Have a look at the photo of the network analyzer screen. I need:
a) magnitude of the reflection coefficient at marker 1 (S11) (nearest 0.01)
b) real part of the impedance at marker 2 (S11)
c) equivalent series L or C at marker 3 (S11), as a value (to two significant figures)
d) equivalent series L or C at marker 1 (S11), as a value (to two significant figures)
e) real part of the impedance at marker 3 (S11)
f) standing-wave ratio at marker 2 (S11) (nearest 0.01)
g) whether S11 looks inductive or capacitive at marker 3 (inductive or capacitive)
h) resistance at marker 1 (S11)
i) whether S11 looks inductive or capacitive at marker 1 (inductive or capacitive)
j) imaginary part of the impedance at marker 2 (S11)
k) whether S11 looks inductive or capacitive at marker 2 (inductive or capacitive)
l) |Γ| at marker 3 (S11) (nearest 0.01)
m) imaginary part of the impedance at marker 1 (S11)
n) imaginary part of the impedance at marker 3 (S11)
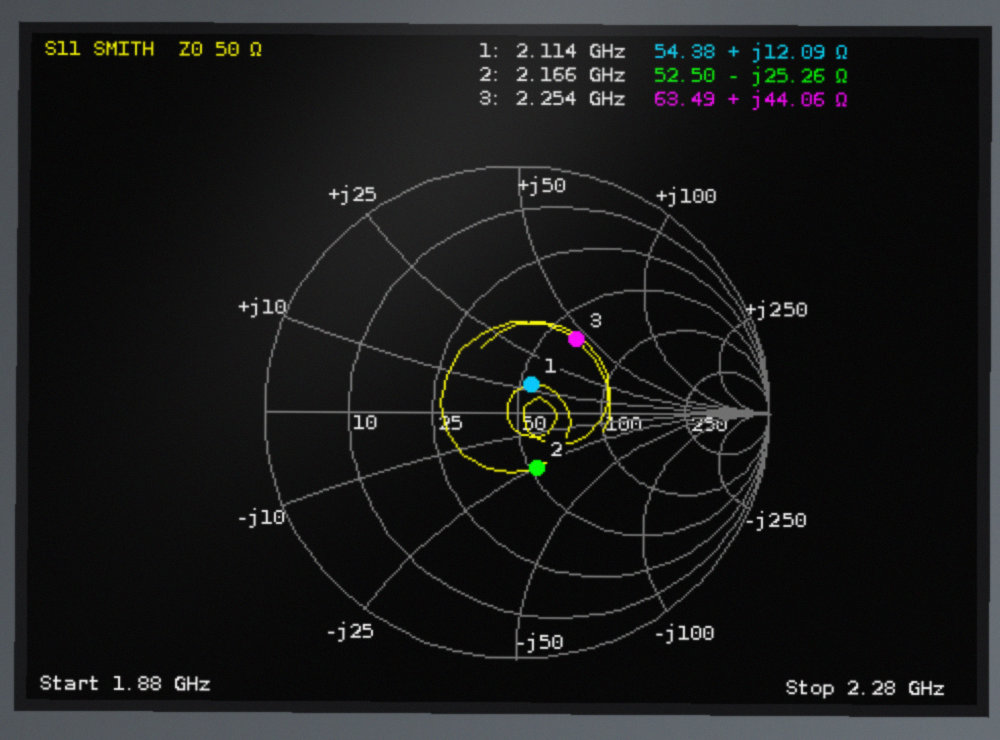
0.12
52.50 Ω
3.1 nH
910 pH
63.49 Ω
1.63
inductive
54.38 Ω
inductive
-25.26 Ω
capacitive
0.38
+12.09 Ω
+44.06 Ω
